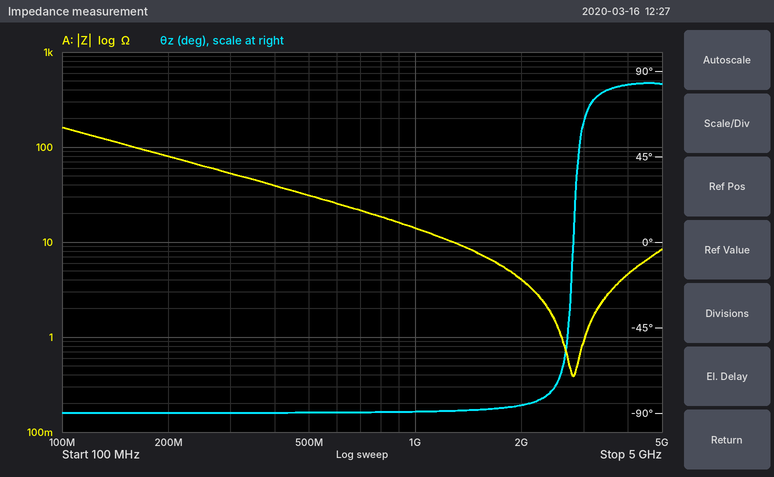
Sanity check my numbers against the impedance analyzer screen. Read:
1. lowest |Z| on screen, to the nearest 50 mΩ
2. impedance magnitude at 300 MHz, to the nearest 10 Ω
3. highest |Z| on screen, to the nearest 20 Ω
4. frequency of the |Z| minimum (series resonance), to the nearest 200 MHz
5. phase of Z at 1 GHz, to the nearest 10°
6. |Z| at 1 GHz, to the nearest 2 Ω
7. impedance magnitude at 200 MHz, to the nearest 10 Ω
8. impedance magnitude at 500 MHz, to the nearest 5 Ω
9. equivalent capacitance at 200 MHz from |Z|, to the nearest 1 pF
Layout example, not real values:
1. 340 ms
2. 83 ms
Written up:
1. 400 mΩ
2. 50 Ω
3. 160 Ω
4. 2.8 GHz
5. -90°
6. 14 Ω
7. 80 Ω
8. 30 Ω
9. 10 pF
